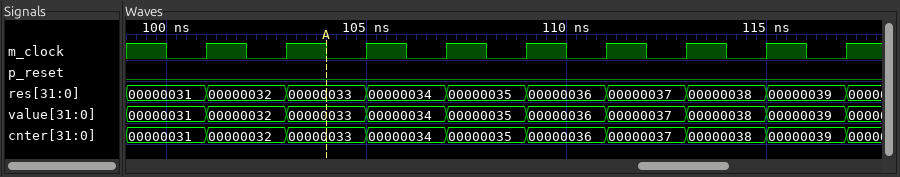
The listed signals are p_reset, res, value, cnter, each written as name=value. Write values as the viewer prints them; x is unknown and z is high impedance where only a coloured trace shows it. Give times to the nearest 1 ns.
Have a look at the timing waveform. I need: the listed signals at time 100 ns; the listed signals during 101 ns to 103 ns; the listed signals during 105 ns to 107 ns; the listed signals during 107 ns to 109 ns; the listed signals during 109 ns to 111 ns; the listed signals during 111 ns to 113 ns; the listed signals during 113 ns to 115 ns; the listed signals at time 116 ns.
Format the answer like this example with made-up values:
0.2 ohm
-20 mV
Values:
p_reset=0, res=00000031, value=00000031, cnter=00000031
p_reset=0, res=00000032, value=00000032, cnter=00000032
p_reset=0, res=00000034, value=00000034, cnter=00000034
p_reset=0, res=00000035, value=00000035, cnter=00000035
p_reset=0, res=00000036, value=00000036, cnter=00000036
p_reset=0, res=00000037, value=00000037, cnter=00000037
p_reset=0, res=00000038, value=00000038, cnter=00000038
p_reset=0, res=00000039, value=00000039, cnter=00000039
